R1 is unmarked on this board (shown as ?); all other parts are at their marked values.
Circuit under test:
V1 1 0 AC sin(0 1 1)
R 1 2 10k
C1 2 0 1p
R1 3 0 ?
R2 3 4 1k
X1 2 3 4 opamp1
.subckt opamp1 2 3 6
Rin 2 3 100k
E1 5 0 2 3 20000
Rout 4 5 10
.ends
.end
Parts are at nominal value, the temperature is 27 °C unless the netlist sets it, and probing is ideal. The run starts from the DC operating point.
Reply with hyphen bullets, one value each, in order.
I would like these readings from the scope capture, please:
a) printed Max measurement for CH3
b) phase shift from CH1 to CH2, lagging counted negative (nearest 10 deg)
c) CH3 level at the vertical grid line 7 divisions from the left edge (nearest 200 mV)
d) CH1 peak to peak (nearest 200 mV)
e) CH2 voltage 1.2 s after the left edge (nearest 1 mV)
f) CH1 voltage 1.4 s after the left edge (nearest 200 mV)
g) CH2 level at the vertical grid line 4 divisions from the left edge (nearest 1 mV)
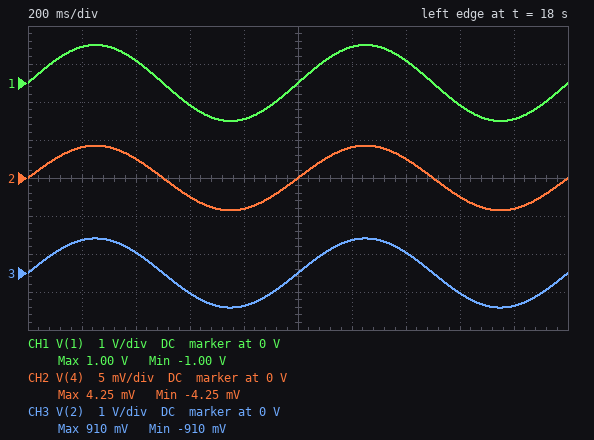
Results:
- 910 mV
- 0 deg
- 600 mV
- 2.0 V
- 4 mV
- 600 mV
- -4 mV
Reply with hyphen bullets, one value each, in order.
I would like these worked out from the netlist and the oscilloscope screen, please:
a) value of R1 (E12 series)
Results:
- 470 Ω
